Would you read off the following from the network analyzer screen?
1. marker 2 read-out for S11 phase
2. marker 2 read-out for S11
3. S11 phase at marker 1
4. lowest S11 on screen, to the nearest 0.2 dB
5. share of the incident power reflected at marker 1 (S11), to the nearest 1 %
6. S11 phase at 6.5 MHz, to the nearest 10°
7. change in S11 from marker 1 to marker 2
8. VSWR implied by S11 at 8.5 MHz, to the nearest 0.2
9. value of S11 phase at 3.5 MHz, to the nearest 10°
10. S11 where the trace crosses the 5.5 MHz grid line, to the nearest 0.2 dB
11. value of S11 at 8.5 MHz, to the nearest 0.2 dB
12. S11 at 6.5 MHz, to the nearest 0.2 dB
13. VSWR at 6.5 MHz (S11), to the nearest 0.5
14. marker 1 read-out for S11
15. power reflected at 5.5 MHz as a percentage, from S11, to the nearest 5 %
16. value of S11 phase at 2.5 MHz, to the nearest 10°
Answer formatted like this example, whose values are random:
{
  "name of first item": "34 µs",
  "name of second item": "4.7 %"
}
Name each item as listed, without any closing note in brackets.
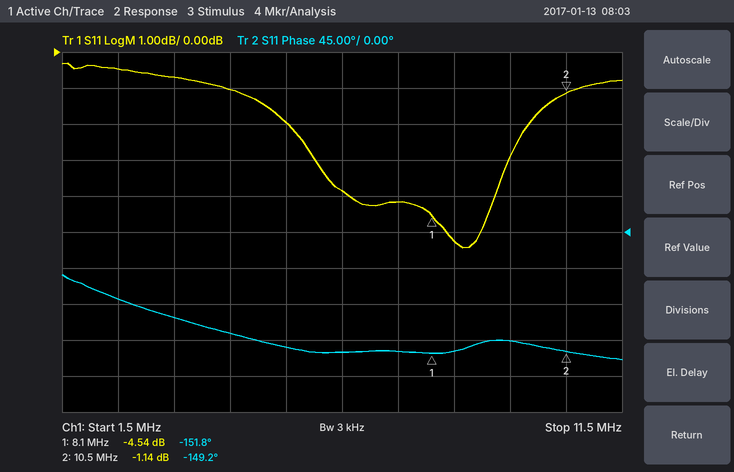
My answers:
{
  "marker 2 read-out for S11 phase": "-149.2°",
  "marker 2 read-out for S11": "-1.14 dB",
  "S11 phase at marker 1": "-151.8°",
  "lowest S11 on screen, to the nearest 0.2 dB": "-5.4 dB",
  "share of the incident power reflected at marker 1 (S11), to the nearest 1 %": "35 %",
  "S11 phase at 6.5 MHz, to the nearest 10°": "-150°",
  "change in S11 from marker 1 to marker 2": "3.40 dB",
  "VSWR implied by S11 at 8.5 MHz, to the nearest 0.2": "3.4",
  "value of S11 phase at 3.5 MHz, to the nearest 10°": "-110°",
  "S11 where the trace crosses the 5.5 MHz grid line, to the nearest 0.2 dB": "-2.0 dB",
  "value of S11 at 8.5 MHz, to the nearest 0.2 dB": "-5.2 dB",
  "S11 at 6.5 MHz, to the nearest 0.2 dB": "-3.8 dB",
  "VSWR at 6.5 MHz (S11), to the nearest 0.5": "4.5",
  "marker 1 read-out for S11": "-4.54 dB",
  "power reflected at 5.5 MHz as a percentage, from S11, to the nearest 5 %": "65 %",
  "value of S11 phase at 2.5 MHz, to the nearest 10°": "-80°"
}
